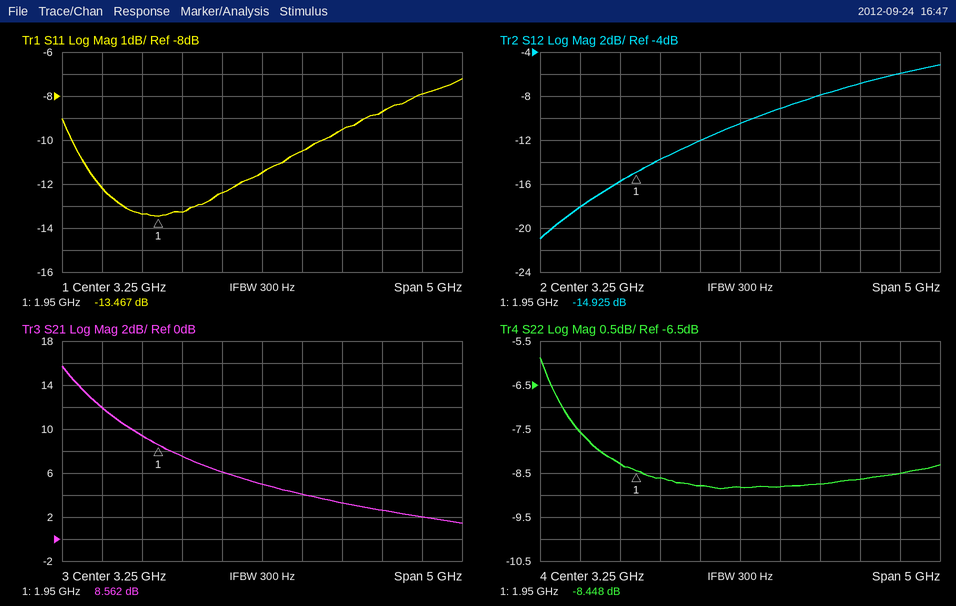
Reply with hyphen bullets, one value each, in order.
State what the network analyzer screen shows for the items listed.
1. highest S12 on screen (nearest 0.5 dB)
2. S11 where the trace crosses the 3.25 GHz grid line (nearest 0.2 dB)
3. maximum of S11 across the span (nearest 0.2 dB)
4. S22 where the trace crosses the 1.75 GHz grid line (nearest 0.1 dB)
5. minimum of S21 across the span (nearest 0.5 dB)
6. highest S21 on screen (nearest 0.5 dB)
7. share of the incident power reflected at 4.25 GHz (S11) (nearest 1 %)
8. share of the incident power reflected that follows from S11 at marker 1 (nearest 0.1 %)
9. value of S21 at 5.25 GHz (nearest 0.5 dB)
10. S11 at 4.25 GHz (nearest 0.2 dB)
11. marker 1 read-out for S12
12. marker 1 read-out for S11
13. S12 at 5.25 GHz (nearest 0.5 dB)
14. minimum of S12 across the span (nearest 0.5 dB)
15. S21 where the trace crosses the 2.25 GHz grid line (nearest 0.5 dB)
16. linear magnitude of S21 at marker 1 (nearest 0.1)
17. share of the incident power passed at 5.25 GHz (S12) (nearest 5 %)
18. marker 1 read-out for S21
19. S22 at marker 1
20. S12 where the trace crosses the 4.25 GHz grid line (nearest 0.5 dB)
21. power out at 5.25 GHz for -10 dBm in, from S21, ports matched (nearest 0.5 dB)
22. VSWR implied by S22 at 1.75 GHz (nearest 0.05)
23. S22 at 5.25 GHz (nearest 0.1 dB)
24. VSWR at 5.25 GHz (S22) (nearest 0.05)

- -5.0 dB
- -11.4 dB
- -7.2 dB
- -8.3 dB
- 1.5 dB
- 15.5 dB
- 11 %
- 4.5 %
- 2.0 dB
- -9.6 dB
- -14.925 dB
- -13.467 dB
- -6.0 dB
- -21.0 dB
- 7.5 dB
- 2.7
- 25 %
- 8.562 dB
- -8.448 dB
- -8.0 dB
- -8.0 dBm
- 2.25
- -8.5 dB
- 2.20
